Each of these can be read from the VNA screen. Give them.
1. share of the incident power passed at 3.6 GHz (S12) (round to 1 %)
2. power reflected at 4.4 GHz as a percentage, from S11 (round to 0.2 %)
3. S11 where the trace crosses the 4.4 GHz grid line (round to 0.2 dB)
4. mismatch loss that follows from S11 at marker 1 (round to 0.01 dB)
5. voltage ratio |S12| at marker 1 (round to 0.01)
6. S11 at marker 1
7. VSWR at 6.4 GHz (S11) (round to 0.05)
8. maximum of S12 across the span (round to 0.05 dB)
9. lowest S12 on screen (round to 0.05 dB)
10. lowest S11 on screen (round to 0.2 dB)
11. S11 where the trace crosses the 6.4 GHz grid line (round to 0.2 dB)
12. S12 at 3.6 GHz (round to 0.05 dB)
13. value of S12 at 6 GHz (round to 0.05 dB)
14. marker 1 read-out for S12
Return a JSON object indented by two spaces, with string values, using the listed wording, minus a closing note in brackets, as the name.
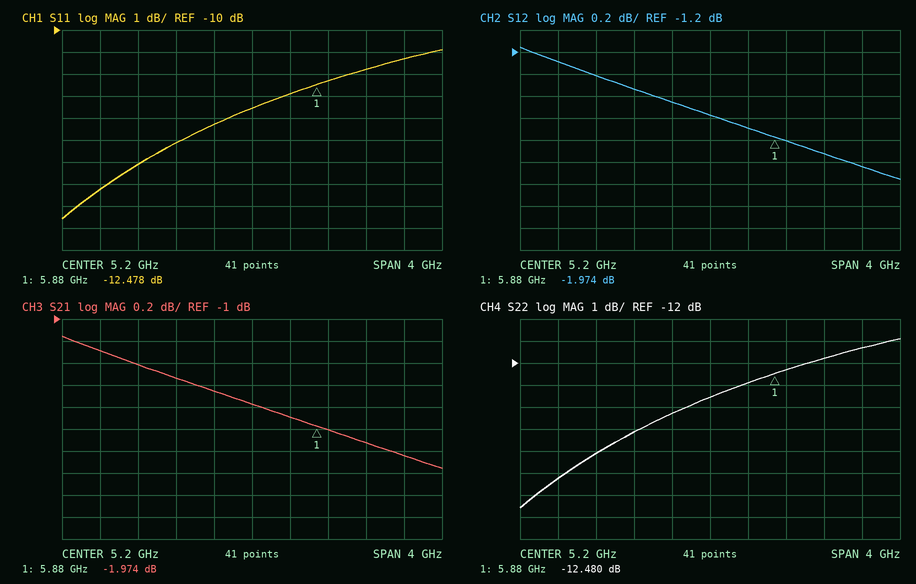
{
  "share of the incident power passed at 3.6 GHz (S12)": "74 %",
  "power reflected at 4.4 GHz as a percentage, from S11": "3.0 %",
  "S11 where the trace crosses the 4.4 GHz grid line": "-15.2 dB",
  "mismatch loss that follows from S11 at marker 1": "0.25 dB",
  "voltage ratio |S12| at marker 1": "0.80",
  "S11 at marker 1": "-12.478 dB",
  "VSWR at 6.4 GHz (S11)": "1.70",
  "maximum of S12 across the span": "-1.15 dB",
  "lowest S12 on screen": "-2.35 dB",
  "lowest S11 on screen": "-18.6 dB",
  "S11 where the trace crosses the 6.4 GHz grid line": "-11.8 dB",
  "S12 at 3.6 GHz": "-1.30 dB",
  "value of S12 at 6 GHz": "-2.00 dB",
  "marker 1 read-out for S12": "-1.974 dB"
}
